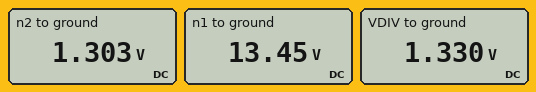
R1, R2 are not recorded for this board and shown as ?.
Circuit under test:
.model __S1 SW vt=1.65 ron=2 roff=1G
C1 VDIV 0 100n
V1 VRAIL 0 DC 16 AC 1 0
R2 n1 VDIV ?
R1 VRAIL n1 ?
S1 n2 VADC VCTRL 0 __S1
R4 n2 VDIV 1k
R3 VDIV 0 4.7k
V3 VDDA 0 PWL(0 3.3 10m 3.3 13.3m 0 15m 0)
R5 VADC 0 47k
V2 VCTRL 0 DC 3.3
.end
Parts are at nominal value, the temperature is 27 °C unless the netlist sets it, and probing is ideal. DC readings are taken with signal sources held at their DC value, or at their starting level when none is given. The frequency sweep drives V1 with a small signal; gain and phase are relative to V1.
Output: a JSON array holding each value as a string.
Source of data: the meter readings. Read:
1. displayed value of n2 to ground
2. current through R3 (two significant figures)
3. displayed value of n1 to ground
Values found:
["1.303 V", "280 µA", "13.45 V"]
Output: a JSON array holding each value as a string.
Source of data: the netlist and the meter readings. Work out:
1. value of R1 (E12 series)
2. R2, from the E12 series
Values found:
["8.2 kΩ", "39 kΩ"]
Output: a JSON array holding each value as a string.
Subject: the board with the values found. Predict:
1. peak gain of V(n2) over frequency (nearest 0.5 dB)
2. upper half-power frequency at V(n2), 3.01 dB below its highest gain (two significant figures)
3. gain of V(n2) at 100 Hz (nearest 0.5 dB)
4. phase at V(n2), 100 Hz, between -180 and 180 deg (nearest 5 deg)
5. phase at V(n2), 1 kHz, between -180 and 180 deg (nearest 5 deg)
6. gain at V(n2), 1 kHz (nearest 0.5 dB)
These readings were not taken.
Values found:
["-21.0 dB", "370 Hz", "-21.0 dB", "-15 deg", "-70 deg", "-30.0 dB"]
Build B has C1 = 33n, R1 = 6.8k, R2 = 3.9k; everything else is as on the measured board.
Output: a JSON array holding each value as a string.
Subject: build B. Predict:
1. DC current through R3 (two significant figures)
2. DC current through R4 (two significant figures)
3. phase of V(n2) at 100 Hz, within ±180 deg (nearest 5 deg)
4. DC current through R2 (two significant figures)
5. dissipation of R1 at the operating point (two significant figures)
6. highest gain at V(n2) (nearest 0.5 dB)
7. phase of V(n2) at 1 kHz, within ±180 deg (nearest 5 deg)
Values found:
["970 µA", "95 µA", "-5 deg", "1.1 mA", "7.8 mW", "-10.5 dB", "-35 deg"]
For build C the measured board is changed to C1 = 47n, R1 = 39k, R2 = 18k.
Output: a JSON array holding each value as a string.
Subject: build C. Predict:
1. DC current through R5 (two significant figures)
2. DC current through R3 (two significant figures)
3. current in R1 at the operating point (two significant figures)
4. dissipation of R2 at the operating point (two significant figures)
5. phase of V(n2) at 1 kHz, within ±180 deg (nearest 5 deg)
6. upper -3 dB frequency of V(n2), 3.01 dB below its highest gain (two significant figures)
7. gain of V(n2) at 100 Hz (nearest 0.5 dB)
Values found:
["23 µA", "240 µA", "260 µA", "1.2 mW", "-50 deg", "780 Hz", "-22.5 dB"]
